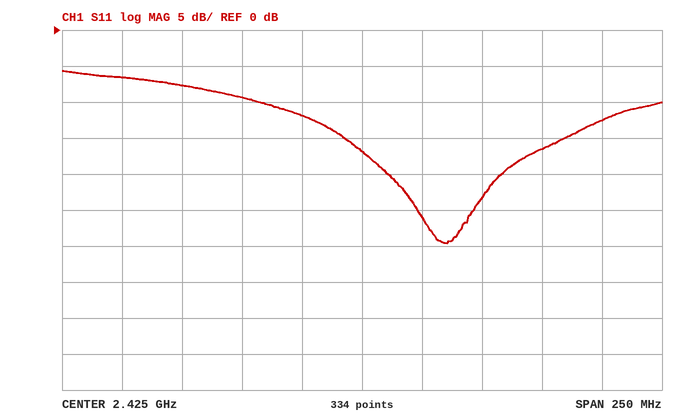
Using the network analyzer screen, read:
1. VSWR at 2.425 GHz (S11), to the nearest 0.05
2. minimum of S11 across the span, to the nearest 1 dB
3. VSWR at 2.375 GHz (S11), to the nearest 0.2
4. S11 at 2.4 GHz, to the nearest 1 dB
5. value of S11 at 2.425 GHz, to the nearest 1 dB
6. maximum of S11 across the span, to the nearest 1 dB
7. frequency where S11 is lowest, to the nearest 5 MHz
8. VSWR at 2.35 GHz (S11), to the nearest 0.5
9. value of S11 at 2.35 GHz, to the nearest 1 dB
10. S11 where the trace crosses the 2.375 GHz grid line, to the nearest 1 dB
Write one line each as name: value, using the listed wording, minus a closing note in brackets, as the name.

VSWR at 2.425 GHz (S11), to the nearest 0.05: 1.35
minimum of S11 across the span, to the nearest 1 dB: -30 dB
VSWR at 2.375 GHz (S11), to the nearest 0.2: 2.0
S11 at 2.4 GHz, to the nearest 1 dB: -12 dB
value of S11 at 2.425 GHz, to the nearest 1 dB: -17 dB
maximum of S11 across the span, to the nearest 1 dB: -6 dB
frequency where S11 is lowest, to the nearest 5 MHz: 2.460 GHz
VSWR at 2.35 GHz (S11), to the nearest 0.5: 2.5
value of S11 at 2.35 GHz, to the nearest 1 dB: -8 dB
S11 where the trace crosses the 2.375 GHz grid line, to the nearest 1 dB: -9 dB
